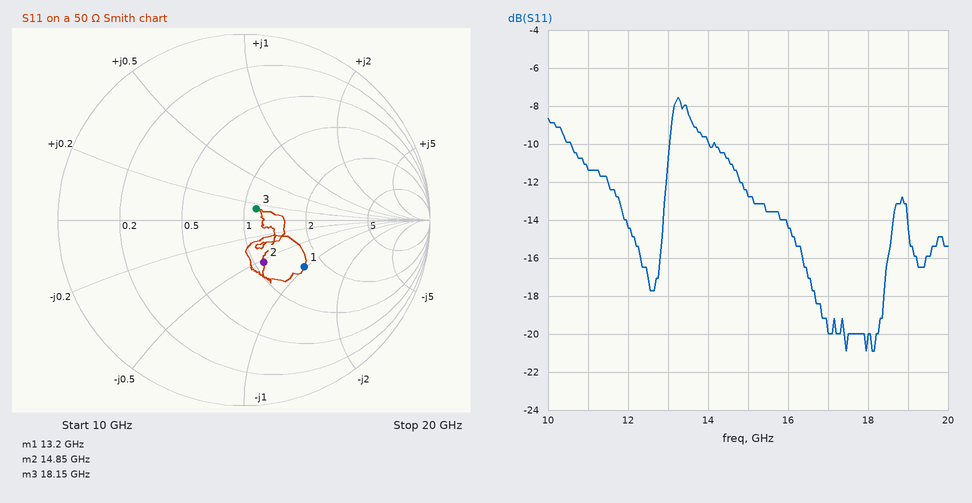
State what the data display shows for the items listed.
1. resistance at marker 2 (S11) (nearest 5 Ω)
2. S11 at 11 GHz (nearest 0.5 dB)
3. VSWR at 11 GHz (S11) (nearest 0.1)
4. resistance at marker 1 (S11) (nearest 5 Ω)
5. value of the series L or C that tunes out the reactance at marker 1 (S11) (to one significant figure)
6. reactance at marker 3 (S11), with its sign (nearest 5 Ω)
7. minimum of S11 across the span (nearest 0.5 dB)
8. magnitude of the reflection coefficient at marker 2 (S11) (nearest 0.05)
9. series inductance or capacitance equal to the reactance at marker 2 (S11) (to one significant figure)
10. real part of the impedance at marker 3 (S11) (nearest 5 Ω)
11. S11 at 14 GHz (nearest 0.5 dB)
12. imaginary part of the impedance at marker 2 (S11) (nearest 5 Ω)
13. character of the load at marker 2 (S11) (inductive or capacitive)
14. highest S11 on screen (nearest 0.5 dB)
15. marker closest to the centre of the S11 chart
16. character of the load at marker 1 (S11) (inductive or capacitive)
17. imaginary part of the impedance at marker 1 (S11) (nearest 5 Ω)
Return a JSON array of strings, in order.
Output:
["55 Ω", "-11.5 dB", "1.7", "80 Ω", "600 pH", "+5 Ω", "-21.0 dB", "0.25", "400 fF", "55 Ω", "-10.0 dB", "-25 Ω", "capacitive", "-7.5 dB", "marker 3", "capacitive", "-50 Ω"]
